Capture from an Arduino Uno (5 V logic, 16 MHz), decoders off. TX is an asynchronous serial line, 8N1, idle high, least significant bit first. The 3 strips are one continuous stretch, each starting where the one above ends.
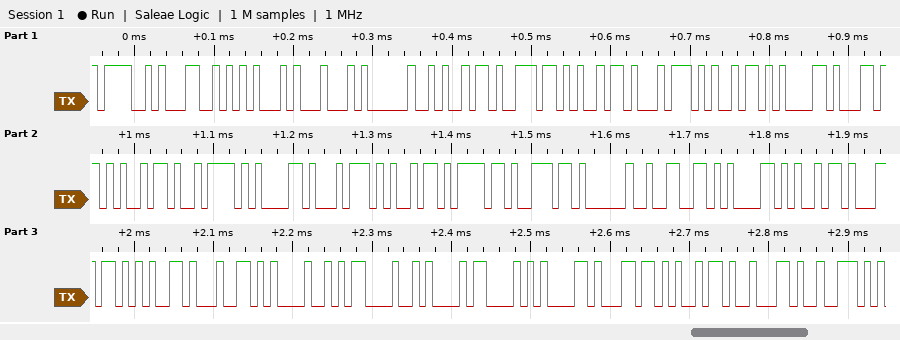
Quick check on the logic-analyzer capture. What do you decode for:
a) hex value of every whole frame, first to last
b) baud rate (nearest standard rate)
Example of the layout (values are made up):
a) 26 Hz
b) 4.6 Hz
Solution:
a) 4F 4C 45 44 20 69 6E 69 74 69 61 6C 69 7A 61 74 69 6F 6E 20 66 61 69 6C 65 64 21 0D 0A 43 61 6C 69 62 72
b) 115200 baud
